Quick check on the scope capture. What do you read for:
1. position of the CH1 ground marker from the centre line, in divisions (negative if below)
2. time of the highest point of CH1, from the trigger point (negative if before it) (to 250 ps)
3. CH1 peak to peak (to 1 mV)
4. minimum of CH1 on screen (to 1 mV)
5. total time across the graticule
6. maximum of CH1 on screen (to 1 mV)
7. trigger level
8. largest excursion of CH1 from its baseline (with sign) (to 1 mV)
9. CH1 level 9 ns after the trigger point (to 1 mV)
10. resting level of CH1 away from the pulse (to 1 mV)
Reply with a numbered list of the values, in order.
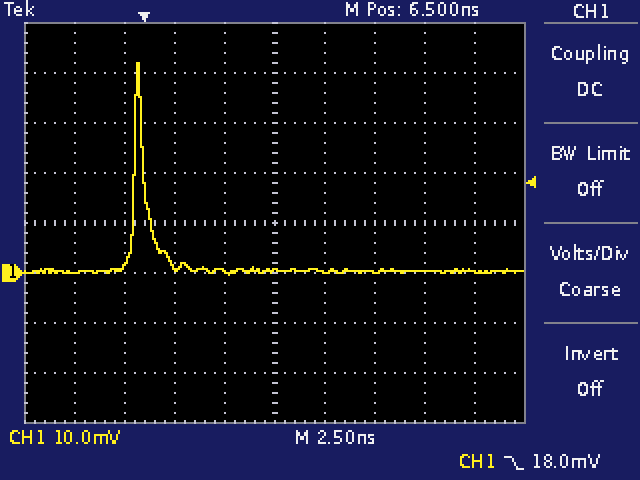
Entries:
1. -1.0 div
2. -250 ps
3. 42 mV
4. 0 mV
5. 25 ns
6. 42 mV
7. 18.0 mV
8. +42 mV
9. 0 mV
10. 0 mV
